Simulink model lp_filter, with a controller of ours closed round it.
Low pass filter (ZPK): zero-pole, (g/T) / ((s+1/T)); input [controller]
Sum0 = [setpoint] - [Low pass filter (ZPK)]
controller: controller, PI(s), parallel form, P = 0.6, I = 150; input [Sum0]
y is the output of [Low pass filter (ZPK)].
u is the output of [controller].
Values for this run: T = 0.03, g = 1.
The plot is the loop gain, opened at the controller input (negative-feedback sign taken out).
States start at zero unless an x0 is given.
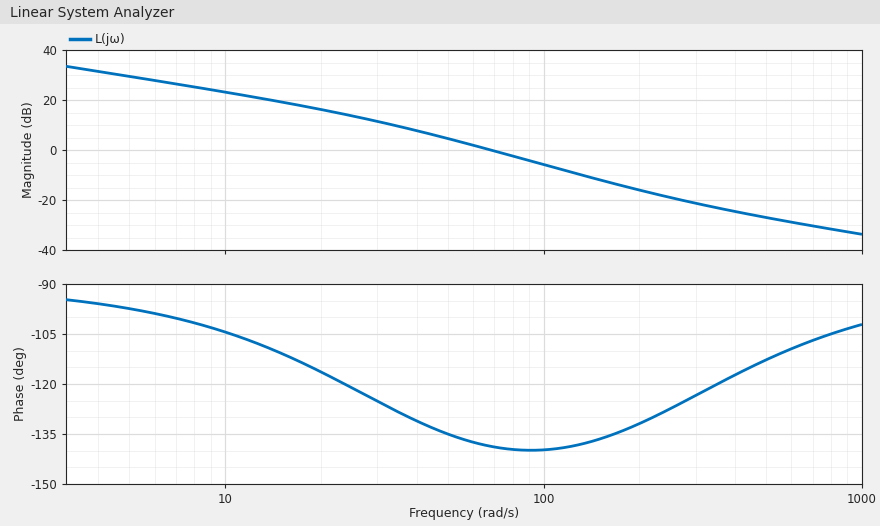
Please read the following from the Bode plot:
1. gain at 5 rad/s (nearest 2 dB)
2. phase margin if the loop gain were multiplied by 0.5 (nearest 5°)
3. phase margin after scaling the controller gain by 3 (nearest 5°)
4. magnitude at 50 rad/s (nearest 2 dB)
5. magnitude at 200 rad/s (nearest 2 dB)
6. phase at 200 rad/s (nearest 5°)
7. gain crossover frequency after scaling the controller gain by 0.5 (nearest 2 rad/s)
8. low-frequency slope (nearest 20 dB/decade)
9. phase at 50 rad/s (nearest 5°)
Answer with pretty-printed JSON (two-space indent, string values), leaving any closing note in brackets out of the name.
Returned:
{
  "gain at 5 rad/s": "30 dB",
  "phase margin if the loop gain were multiplied by 0.5": "45°",
  "phase margin after scaling the controller gain by 3": "40°",
  "magnitude at 50 rad/s": "4 dB",
  "magnitude at 200 rad/s": "-16 dB",
  "phase at 200 rad/s": "-130°",
  "gain crossover frequency after scaling the controller gain by 0.5": "46 rad/s",
  "low-frequency slope": "-20 dB/decade",
  "phase at 50 rad/s": "-135°"
}
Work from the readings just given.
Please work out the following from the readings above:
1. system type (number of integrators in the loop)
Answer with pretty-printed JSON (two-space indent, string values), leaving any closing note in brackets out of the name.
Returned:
{
  "system type": "1"
}
